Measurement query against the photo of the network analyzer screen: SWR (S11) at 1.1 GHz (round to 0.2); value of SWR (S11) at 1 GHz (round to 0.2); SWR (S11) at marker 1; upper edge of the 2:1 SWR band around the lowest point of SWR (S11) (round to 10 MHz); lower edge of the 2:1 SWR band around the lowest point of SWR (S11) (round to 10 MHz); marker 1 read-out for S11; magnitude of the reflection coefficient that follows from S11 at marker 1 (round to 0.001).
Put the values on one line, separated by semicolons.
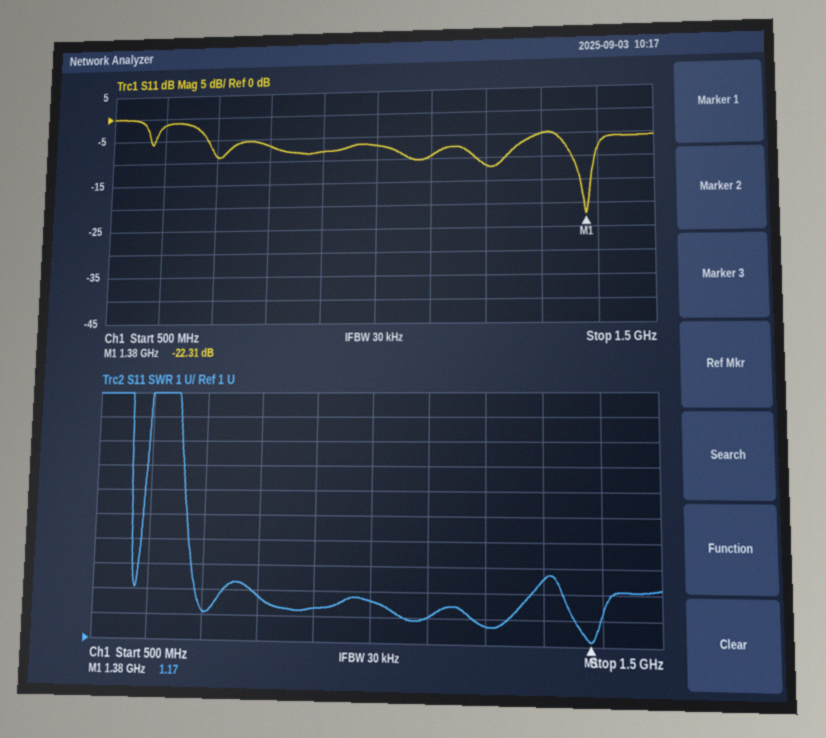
2.0; 2.6; 1.17; 1.40 GHz; 1.35 GHz; -22.31 dB; 0.077
